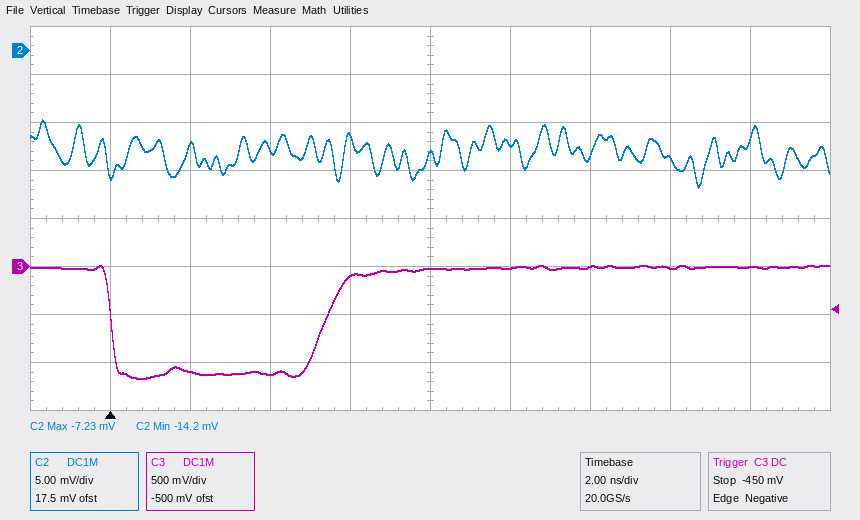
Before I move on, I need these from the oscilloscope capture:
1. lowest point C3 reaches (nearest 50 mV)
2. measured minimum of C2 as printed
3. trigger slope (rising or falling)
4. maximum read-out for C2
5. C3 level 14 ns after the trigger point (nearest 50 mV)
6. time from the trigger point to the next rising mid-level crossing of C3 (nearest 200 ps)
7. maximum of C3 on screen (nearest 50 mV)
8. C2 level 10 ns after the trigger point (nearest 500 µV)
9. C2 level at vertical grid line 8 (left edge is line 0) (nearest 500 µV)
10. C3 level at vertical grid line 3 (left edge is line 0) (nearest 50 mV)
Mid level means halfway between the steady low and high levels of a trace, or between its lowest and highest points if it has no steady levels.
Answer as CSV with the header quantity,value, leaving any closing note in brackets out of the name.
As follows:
quantity,value
lowest point C3 reaches,-1.15 V
measured minimum of C2 as printed,-14.2 mV
trigger slope,falling
maximum read-out for C2,-7.23 mV
C3 level 14 ns after the trigger point,0 mV
time from the trigger point to the next rising mid-level crossing of C3,5.4 ns
maximum of C3 on screen,0 mV
C2 level 10 ns after the trigger point,-9.5 mV
C2 level at vertical grid line 8 (left edge is line 0),-11.5 mV
C3 level at vertical grid line 3 (left edge is line 0),-1.10 V
